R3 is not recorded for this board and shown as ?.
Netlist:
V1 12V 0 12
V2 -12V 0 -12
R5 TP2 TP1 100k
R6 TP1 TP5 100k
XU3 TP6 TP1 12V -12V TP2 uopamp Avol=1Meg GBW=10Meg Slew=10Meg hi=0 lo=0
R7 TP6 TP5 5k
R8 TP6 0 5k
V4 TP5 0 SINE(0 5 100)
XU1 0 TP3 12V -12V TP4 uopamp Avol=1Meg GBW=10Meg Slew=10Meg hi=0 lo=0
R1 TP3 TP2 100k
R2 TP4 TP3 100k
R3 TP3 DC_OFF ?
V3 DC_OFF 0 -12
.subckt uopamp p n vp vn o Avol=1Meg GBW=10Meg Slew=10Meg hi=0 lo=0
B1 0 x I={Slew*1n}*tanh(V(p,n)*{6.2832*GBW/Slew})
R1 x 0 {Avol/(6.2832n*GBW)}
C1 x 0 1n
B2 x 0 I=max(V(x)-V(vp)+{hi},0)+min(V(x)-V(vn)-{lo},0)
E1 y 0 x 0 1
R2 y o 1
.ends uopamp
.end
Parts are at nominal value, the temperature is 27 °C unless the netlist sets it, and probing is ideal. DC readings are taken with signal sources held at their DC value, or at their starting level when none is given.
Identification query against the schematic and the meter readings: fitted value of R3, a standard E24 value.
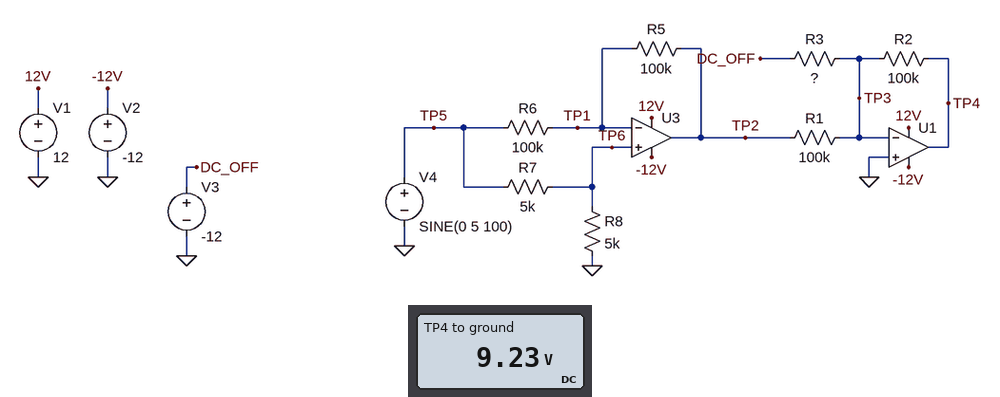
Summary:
130 kΩ
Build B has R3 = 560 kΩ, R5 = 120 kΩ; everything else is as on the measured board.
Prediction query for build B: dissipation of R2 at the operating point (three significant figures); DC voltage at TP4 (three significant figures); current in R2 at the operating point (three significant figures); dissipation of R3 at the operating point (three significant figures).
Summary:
45.9 µW
2.14 V
21.4 µA
257 µW
